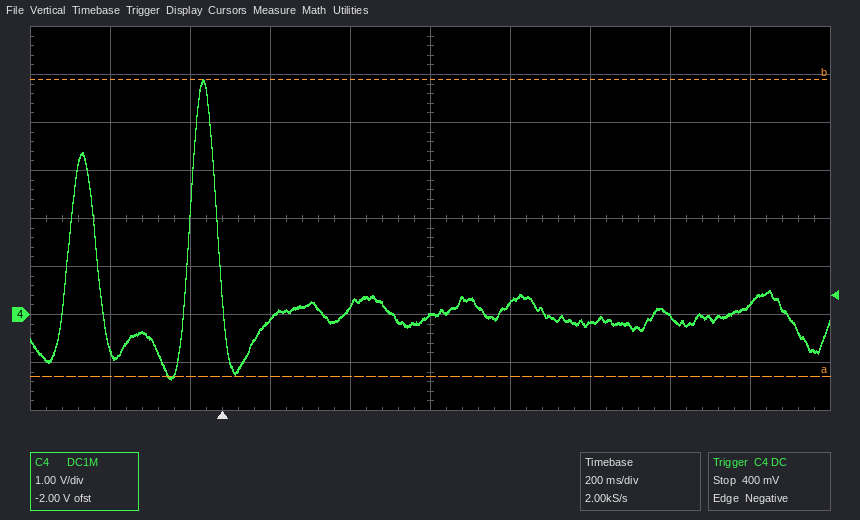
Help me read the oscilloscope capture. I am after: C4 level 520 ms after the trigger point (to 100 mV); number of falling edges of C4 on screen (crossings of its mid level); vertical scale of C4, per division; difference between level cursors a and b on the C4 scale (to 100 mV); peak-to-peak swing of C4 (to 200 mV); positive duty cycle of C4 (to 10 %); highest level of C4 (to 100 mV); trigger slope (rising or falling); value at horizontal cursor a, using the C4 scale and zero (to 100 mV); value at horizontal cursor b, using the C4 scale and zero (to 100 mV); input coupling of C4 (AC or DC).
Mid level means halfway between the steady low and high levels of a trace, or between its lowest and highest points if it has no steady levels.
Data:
0.0 V
2
1 V
6.2 V
6.2 V
20 %
4.9 V
falling
-1.3 V
4.9 V
DC
